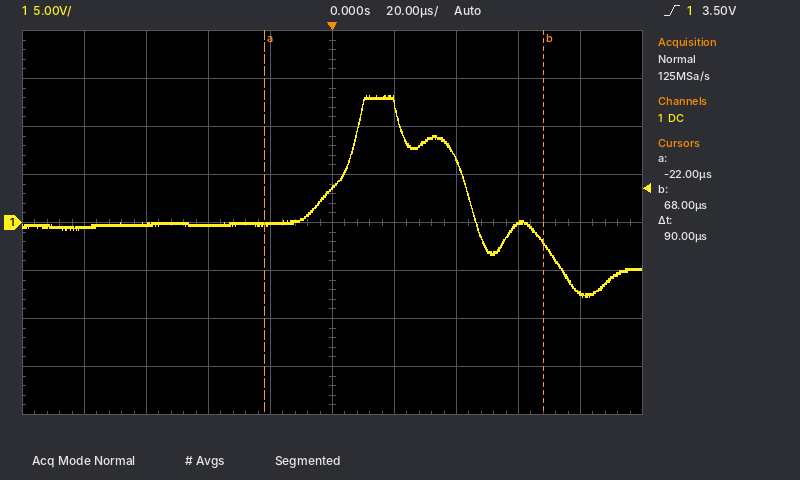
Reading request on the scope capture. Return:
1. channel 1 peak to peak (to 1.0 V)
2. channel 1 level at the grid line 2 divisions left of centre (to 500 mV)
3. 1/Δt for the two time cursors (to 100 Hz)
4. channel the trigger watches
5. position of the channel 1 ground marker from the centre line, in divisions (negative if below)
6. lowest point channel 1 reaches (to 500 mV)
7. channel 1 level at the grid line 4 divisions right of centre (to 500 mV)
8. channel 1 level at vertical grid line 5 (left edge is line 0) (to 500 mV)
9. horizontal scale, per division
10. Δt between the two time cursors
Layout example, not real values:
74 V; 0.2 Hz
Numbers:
21.0 V; -500 mV; 11.1 kHz; channel 1; 0.0 div; -8.0 V; -7.5 V; 3.5 V; 20 µs; 90 µs
